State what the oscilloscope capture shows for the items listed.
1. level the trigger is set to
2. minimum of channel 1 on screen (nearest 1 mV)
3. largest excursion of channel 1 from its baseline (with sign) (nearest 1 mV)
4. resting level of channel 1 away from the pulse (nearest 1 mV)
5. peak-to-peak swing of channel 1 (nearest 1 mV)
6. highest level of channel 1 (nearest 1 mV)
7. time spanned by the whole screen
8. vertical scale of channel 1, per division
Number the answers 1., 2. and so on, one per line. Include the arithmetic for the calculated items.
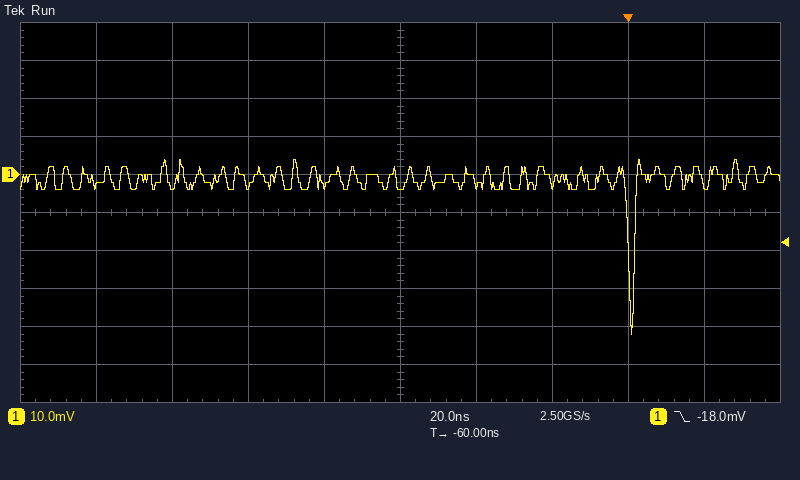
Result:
1. -18.0 mV
2. -42 mV
3. -42 mV − (-1 mV) = -41 mV
4. -1 mV
5. 4 mV − (-42 mV) = 46 mV
6. 4 mV
7. 200 ns
8. 10 mV
